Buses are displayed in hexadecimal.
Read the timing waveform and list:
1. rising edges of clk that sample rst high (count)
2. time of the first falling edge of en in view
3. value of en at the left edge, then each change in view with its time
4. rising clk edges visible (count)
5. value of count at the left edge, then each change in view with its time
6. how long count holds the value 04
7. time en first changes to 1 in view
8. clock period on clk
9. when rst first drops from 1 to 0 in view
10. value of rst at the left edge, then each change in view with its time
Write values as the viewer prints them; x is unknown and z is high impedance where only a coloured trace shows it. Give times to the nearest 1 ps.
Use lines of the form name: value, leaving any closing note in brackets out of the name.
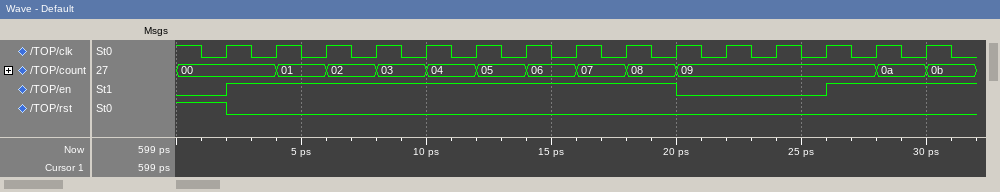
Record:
rising edges of clk that sample rst high: 1
time of the first falling edge of en in view: 20 ps
value of en at the left edge, then each change in view with its time: 0, 1 at 2 ps, 0 at 20 ps, 1 at 26 ps
rising clk edges visible: 15
value of count at the left edge, then each change in view with its time: 00, 01 at 4 ps, 02 at 6 ps, 03 at 8 ps, 04 at 10 ps, 05 at 12 ps, 06 at 14 ps, 07 at 16 ps, 08 at 18 ps, 09 at 20 ps, 0a at 28 ps, 0b at 30 ps
how long count holds the value 04: 2 ps
time en first changes to 1 in view: 2 ps
clock period on clk: 2 ps
when rst first drops from 1 to 0 in view: 2 ps
value of rst at the left edge, then each change in view with its time: 1, 0 at 2 ps
